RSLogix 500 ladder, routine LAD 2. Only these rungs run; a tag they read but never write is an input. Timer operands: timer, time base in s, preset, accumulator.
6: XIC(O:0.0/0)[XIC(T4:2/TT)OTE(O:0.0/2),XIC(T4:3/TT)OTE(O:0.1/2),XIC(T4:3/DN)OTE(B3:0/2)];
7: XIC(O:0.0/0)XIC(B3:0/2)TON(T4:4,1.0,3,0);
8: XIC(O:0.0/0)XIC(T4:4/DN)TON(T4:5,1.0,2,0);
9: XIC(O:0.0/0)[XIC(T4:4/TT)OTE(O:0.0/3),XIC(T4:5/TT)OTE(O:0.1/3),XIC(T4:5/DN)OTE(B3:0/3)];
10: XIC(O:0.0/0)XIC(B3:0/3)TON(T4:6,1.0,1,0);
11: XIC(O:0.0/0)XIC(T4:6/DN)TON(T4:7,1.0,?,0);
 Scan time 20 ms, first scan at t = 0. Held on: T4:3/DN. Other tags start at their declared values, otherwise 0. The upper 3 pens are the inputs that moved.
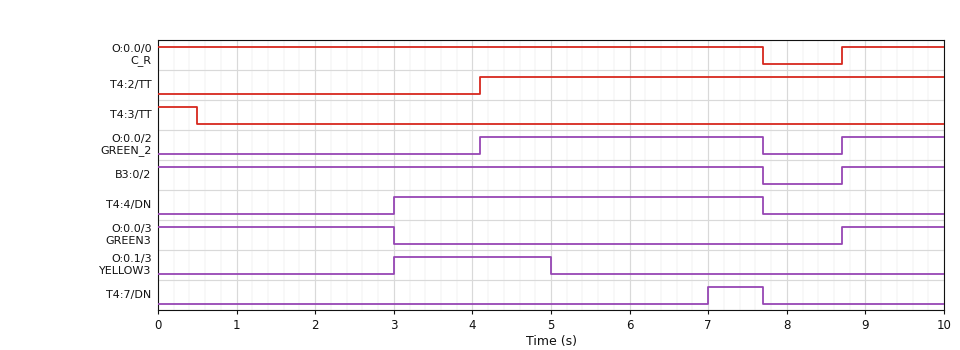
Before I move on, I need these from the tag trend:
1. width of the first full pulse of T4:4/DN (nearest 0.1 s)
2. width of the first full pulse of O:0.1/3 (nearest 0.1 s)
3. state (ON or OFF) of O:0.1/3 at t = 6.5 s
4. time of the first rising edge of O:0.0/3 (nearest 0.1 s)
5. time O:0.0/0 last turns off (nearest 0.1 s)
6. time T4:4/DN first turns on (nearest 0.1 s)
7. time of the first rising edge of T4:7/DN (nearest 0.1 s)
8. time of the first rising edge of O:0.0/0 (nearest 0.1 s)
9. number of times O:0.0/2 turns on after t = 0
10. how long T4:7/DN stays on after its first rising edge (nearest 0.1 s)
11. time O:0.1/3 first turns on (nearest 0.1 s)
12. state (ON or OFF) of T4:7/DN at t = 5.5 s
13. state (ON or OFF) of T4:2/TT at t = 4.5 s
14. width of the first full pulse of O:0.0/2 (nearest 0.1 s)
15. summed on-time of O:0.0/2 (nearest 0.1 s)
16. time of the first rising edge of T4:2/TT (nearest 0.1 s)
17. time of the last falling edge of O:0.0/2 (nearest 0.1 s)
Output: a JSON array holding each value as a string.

["4.7 s", "2.0 s", "OFF", "8.7 s", "7.7 s", "3.0 s", "7.0 s", "8.7 s", "2", "0.7 s", "3.0 s", "OFF", "ON", "3.6 s", "4.9 s", "4.1 s", "7.7 s"]
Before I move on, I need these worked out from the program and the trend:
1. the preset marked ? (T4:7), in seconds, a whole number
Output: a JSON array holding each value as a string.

["1 s"]
